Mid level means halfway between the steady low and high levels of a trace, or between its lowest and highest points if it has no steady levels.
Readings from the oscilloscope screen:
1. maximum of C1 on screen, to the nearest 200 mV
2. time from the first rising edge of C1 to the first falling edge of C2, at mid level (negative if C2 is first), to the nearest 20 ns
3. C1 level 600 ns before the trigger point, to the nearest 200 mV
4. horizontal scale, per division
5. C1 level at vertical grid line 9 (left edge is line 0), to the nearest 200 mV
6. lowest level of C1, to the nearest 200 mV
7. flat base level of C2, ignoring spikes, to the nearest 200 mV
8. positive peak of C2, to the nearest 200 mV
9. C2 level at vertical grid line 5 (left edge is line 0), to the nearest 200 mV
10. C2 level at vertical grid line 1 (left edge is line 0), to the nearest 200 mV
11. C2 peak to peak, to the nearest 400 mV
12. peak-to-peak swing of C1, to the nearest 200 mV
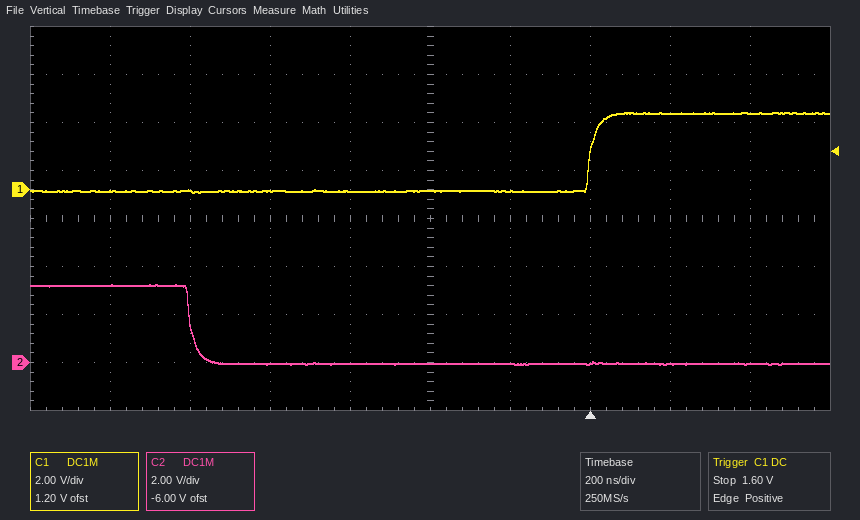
3.2 V
-1.00 µs
0.0 V
200 ns
3.2 V
-200 mV
0.0 V
3.2 V
0.0 V
3.2 V
3.2 V
3.4 V
